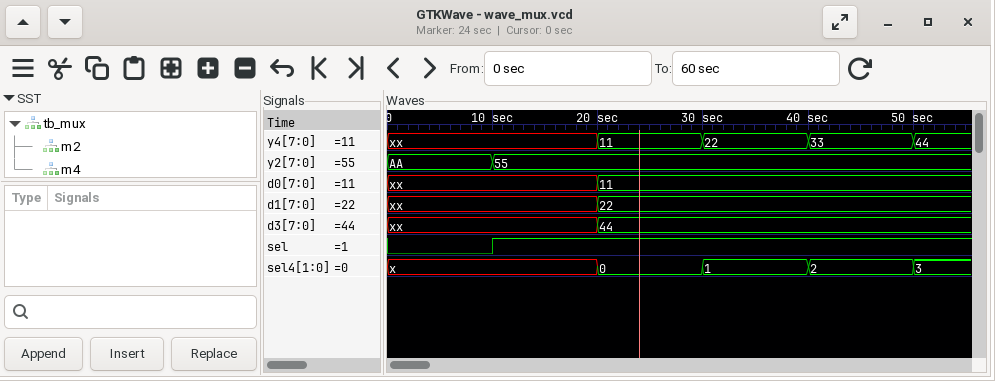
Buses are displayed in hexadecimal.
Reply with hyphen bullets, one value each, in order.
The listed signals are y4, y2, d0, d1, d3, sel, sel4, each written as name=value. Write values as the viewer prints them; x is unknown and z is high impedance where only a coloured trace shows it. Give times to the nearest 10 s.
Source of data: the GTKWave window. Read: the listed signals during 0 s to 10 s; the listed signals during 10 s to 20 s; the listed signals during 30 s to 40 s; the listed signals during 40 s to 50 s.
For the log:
- y4=xx, y2=AA, d0=xx, d1=xx, d3=xx, sel=0, sel4=x
- y4=xx, y2=55, d0=xx, d1=xx, d3=xx, sel=1, sel4=x
- y4=22, y2=55, d0=11, d1=22, d3=44, sel=1, sel4=1
- y4=33, y2=55, d0=11, d1=22, d3=44, sel=1, sel4=2
